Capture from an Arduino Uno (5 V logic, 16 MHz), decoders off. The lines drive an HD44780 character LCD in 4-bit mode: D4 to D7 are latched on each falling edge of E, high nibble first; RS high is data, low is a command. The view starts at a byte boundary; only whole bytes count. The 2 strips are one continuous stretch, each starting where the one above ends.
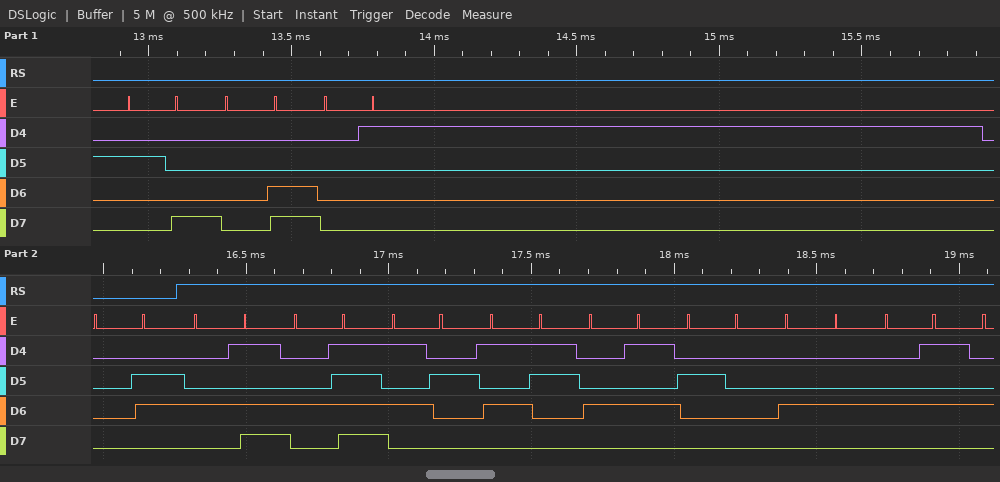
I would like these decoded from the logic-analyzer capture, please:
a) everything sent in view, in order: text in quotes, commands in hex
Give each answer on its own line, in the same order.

0x28 0x0C 0x01 0x06 "MORSE DE"
